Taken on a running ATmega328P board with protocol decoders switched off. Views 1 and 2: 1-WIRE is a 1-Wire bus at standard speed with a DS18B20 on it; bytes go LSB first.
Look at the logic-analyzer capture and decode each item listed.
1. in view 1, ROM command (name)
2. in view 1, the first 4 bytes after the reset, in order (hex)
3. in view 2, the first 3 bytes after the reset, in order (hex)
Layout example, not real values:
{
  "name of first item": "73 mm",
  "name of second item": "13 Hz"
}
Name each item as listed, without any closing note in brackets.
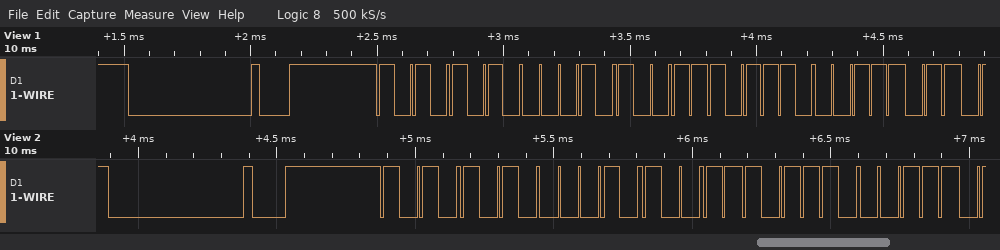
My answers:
{
  "in view 1, ROM command": "Match ROM",
  "in view 1, the first 4 bytes after the reset, in order": "55 28 77 DC",
  "in view 2, the first 3 bytes after the reset, in order": "55 28 77"
}
